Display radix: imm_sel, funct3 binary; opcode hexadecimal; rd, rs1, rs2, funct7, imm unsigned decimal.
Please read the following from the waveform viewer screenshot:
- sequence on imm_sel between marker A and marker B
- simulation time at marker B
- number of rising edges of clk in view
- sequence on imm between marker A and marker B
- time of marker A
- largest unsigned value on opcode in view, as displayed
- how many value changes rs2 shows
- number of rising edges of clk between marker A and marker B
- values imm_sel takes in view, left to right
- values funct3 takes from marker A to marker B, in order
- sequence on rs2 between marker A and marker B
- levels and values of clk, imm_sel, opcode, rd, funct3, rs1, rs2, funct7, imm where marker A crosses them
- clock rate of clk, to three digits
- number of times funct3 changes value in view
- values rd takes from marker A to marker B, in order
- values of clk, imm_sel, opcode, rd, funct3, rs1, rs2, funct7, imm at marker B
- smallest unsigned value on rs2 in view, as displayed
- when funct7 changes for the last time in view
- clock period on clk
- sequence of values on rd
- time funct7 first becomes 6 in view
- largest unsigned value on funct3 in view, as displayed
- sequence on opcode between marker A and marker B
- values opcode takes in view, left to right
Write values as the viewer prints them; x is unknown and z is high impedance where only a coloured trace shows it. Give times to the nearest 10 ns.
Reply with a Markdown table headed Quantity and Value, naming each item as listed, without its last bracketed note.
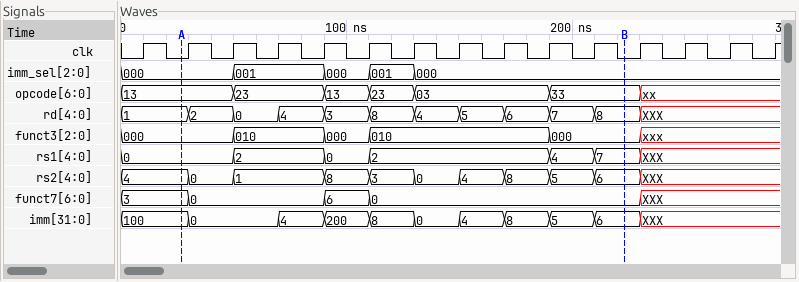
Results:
| Quantity | Value |
|---|---|
| sequence on imm_sel between marker A and marker B | 000, 001, 000, 001, 000 |
| simulation time at marker B | 220 ns |
| number of rising edges of clk in view | 15 |
| sequence on imm between marker A and marker B | 100, 0, 4, 200, 8, 0, 4, 8, 5, 6 |
| time of marker A | 30 ns |
| largest unsigned value on opcode in view, as displayed | 33 |
| how many value changes rs2 shows | 10 |
| number of rising edges of clk between marker A and marker B | 10 |
| values imm_sel takes in view, left to right | 000, 001, 000, 001, 000 |
| values funct3 takes from marker A to marker B, in order | 000, 010, 000, 010, 000 |
| sequence on rs2 between marker A and marker B | 4, 0, 1, 8, 3, 0, 4, 8, 5, 6 |
| levels and values of clk, imm_sel, opcode, rd, funct3, rs1, rs2, funct7, imm where marker A crosses them | clk=0, imm_sel=000, opcode=13, rd=1, funct3=000, rs1=0, rs2=4, funct7=3, imm=100 |
| clock rate of clk, to three digits | 50.0 MHz |
| number of times funct3 changes value in view | 5 |
| values rd takes from marker A to marker B, in order | 1, 2, 0, 4, 3, 8, 4, 5, 6, 7, 8 |
| values of clk, imm_sel, opcode, rd, funct3, rs1, rs2, funct7, imm at marker B | clk=0, imm_sel=000, opcode=33, rd=8, funct3=000, rs1=7, rs2=6, funct7=0, imm=6 |
| smallest unsigned value on rs2 in view, as displayed | 0 |
| when funct7 changes for the last time in view | 230 ns |
| clock period on clk | 20 ns |
| sequence of values on rd | 1, 2, 0, 4, 3, 8, 4, 5, 6, 7, 8, XXX |
| time funct7 first becomes 6 in view | 90 ns |
| largest unsigned value on funct3 in view, as displayed | 010 |
| sequence on opcode between marker A and marker B | 13, 23, 13, 23, 03, 33 |
| values opcode takes in view, left to right | 13, 23, 13, 23, 03, 33, xx |
